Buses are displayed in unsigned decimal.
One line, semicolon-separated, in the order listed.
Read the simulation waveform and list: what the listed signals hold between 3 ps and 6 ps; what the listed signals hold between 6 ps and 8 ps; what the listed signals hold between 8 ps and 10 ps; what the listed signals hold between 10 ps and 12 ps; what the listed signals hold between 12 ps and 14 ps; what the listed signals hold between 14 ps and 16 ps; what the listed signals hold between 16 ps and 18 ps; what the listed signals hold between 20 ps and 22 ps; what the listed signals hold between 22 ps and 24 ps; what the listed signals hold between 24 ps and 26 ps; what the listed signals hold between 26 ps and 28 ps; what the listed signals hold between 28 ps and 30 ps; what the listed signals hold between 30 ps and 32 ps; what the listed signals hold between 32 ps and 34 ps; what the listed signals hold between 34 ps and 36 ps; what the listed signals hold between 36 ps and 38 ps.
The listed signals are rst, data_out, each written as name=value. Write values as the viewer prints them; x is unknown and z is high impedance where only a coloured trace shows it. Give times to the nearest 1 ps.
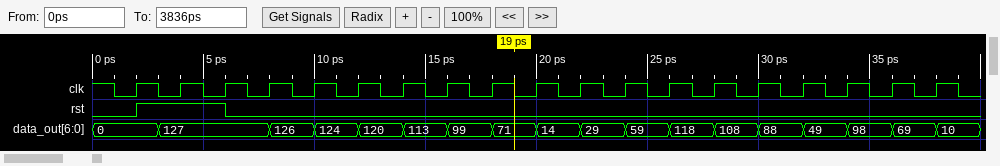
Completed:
rst=1, data_out=127; rst=0, data_out=127; rst=0, data_out=126; rst=0, data_out=124; rst=0, data_out=120; rst=0, data_out=113; rst=0, data_out=99; rst=0, data_out=14; rst=0, data_out=29; rst=0, data_out=59; rst=0, data_out=118; rst=0, data_out=108; rst=0, data_out=88; rst=0, data_out=49; rst=0, data_out=98; rst=0, data_out=69
